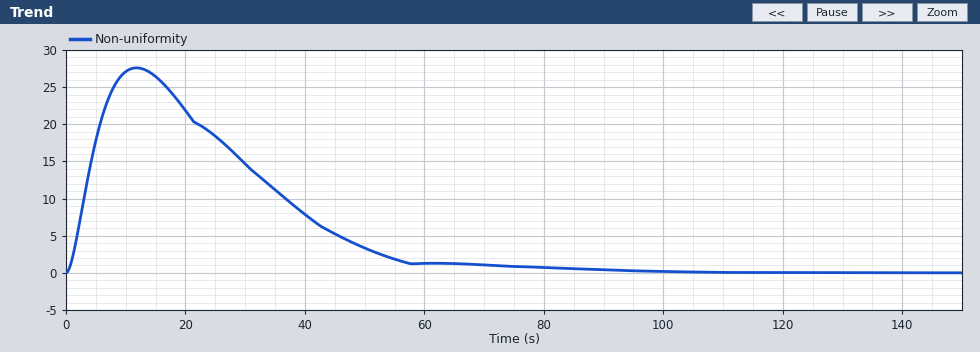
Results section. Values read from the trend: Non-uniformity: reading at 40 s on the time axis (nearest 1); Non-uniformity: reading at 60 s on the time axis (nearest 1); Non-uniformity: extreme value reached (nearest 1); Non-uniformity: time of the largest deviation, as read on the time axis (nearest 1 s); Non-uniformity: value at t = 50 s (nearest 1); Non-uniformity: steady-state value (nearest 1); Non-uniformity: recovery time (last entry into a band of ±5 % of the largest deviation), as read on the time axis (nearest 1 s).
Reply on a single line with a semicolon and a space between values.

8; 1; 28; 12 s; 3; 0; 57 s
